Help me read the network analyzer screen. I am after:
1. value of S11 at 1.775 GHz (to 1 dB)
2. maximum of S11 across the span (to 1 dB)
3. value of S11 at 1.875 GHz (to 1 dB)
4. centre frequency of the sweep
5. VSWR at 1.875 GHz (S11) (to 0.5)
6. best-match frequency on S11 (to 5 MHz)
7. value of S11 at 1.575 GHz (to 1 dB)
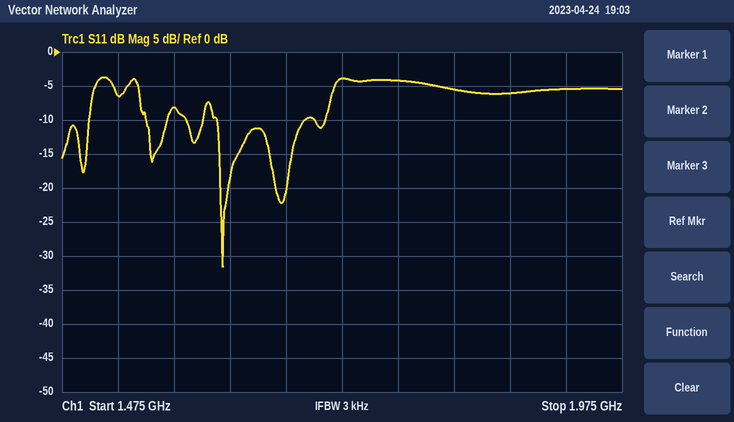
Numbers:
-4 dB
-4 dB
-6 dB
1.725 GHz
3.0
1.620 GHz
-8 dB
